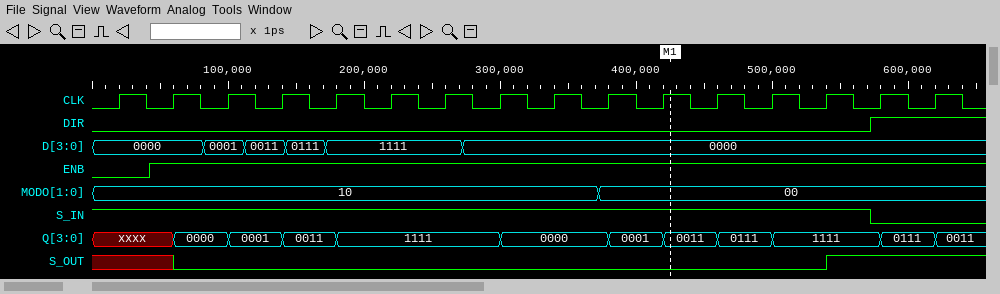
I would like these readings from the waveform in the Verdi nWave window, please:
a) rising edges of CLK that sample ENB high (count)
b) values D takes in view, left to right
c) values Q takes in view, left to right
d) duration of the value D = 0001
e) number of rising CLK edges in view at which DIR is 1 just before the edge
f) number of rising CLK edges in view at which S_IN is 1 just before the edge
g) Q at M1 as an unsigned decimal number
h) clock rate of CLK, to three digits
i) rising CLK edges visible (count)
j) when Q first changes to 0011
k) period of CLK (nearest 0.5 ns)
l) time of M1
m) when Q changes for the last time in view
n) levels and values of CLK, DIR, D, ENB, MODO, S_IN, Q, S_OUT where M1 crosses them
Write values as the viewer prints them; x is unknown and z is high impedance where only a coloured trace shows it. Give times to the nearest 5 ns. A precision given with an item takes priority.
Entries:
15
0000, 0001, 0011, 0111, 1111, 0000
xxxx, 0000, 0001, 0011, 1111, 0000, 0001, 0011, 0111, 1111, 0111, 0011
30 ns
2
14
3
25.0 MHz
16
140 ns
40 ns
425 ns
620 ns
CLK=1, DIR=0, D=0000, ENB=1, MODO=00, S_IN=1, Q=0011, S_OUT=0
